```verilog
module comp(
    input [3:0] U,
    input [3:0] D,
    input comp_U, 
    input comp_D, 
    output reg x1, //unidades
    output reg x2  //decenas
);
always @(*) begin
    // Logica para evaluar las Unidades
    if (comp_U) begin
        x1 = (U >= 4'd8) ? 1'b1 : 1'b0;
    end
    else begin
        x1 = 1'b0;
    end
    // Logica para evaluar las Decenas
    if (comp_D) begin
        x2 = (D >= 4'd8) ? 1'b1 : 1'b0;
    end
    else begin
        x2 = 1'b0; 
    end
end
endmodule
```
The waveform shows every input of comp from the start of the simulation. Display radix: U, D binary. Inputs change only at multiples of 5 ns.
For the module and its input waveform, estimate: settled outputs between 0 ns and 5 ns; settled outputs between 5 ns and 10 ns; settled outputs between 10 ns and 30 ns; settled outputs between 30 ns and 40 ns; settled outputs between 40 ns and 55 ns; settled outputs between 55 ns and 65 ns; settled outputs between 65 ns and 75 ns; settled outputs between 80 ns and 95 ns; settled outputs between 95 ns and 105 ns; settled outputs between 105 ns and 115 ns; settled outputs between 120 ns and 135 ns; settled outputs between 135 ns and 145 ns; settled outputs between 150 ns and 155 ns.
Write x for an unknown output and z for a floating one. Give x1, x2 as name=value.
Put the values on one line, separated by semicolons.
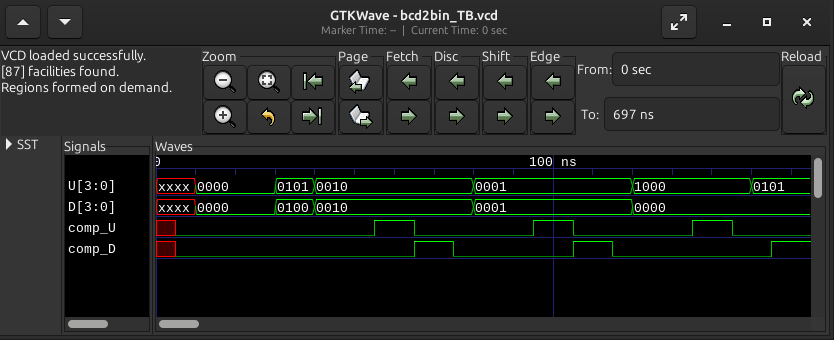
x1=x, x2=x; x1=0, x2=0; x1=0, x2=0; x1=0, x2=0; x1=0, x2=0; x1=0, x2=0; x1=0, x2=0; x1=0, x2=0; x1=0, x2=0; x1=0, x2=0; x1=0, x2=0; x1=1, x2=0; x1=0, x2=0
